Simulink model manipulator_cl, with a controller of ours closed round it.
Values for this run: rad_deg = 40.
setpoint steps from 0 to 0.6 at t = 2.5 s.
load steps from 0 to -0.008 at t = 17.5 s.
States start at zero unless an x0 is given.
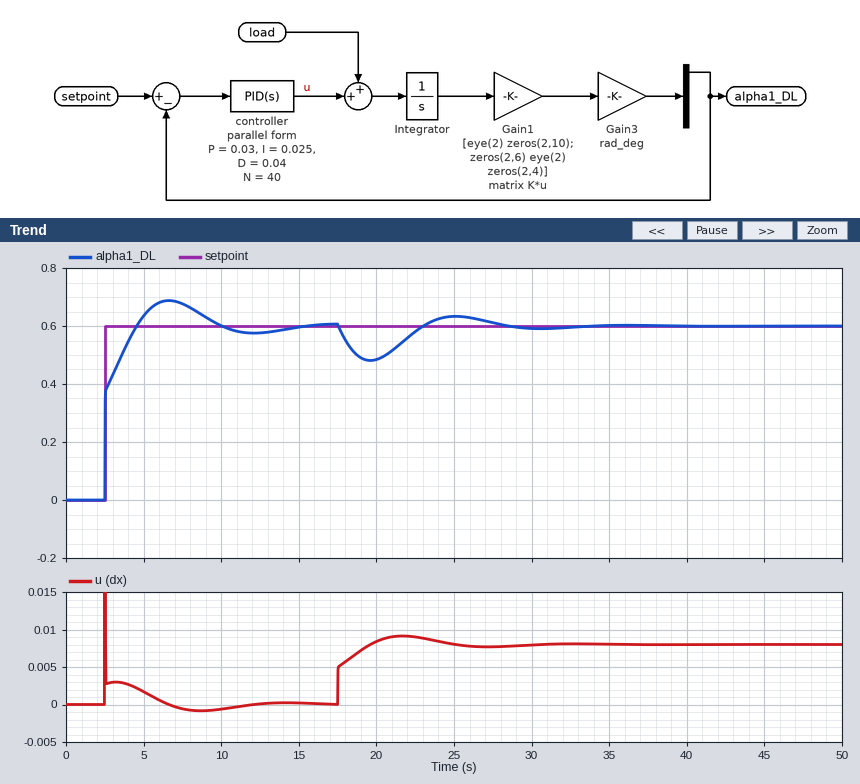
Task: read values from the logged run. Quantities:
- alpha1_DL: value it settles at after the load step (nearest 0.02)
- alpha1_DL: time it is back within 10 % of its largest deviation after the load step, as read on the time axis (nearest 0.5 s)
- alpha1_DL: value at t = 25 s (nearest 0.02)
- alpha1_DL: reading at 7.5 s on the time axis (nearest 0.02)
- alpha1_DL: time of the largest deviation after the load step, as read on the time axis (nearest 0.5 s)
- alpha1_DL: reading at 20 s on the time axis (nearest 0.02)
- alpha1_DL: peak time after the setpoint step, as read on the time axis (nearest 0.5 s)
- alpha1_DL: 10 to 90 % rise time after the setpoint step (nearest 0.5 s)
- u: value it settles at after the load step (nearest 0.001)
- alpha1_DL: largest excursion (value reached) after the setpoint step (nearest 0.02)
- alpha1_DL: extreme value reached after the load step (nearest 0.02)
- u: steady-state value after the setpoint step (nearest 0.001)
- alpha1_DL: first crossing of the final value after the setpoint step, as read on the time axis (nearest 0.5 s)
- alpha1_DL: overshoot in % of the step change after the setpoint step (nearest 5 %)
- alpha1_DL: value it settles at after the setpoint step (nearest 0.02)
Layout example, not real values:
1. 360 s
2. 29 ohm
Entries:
1. 0.60
2. 27.5 s
3. 0.64
4. 0.68
5. 19.5 s
6. 0.48
7. 6.5 s
8. 1.5 s
9. 0.008
10. 0.68
11. 0.48
12. 0.000
13. 4.5 s
14. 15 %
15. 0.60
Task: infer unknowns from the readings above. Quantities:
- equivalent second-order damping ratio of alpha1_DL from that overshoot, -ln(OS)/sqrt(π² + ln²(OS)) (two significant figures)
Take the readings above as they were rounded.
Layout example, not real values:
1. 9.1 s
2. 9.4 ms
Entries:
1. 0.52
